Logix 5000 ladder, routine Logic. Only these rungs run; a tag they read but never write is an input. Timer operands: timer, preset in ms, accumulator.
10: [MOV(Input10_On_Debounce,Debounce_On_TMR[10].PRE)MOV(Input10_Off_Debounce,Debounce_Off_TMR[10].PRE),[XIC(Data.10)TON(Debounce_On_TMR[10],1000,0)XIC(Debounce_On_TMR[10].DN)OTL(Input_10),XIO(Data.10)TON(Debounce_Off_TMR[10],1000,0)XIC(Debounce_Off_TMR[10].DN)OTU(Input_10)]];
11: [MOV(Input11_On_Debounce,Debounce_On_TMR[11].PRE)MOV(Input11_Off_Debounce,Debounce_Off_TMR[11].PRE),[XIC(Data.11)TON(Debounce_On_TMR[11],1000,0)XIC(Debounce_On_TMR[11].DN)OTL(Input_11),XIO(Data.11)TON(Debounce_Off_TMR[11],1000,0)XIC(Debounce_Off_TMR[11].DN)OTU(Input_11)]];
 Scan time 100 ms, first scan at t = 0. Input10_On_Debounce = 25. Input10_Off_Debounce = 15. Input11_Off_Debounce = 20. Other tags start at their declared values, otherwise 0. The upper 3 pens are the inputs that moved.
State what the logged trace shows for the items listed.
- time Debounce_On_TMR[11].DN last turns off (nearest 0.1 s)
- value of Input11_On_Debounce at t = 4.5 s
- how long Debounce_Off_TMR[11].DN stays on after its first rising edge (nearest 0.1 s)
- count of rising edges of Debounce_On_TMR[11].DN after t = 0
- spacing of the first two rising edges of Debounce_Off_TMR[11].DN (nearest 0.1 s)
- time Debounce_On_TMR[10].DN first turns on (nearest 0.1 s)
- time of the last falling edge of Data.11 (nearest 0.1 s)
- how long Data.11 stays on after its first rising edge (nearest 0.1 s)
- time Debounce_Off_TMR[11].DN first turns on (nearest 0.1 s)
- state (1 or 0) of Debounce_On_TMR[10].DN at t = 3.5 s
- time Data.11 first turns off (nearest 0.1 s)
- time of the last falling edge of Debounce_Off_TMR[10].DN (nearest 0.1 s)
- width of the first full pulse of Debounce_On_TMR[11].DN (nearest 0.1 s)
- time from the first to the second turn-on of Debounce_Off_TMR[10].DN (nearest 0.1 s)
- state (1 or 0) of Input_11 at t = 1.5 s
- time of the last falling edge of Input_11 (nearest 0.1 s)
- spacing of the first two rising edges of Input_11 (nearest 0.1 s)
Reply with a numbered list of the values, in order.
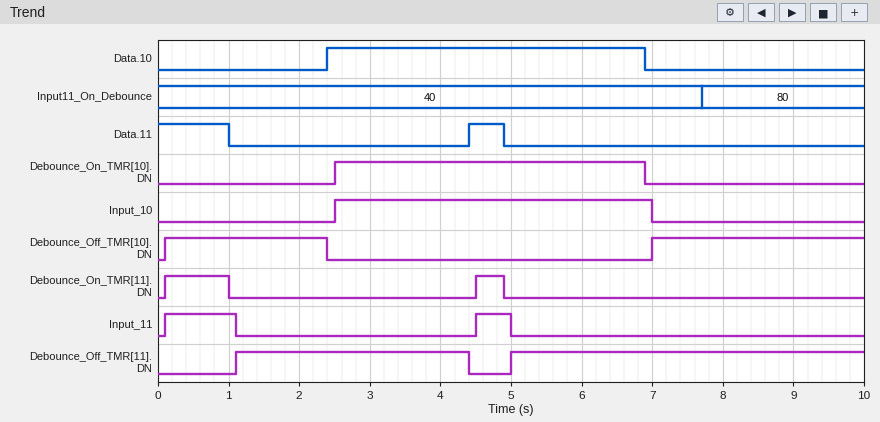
1. 4.9 s
2. 40
3. 3.3 s
4. 2
5. 3.9 s
6. 2.5 s
7. 4.9 s
8. 0.5 s
9. 1.1 s
10. 1
11. 1.0 s
12. 2.4 s
13. 0.9 s
14. 6.9 s
15. 0
16. 5.0 s
17. 4.4 s
